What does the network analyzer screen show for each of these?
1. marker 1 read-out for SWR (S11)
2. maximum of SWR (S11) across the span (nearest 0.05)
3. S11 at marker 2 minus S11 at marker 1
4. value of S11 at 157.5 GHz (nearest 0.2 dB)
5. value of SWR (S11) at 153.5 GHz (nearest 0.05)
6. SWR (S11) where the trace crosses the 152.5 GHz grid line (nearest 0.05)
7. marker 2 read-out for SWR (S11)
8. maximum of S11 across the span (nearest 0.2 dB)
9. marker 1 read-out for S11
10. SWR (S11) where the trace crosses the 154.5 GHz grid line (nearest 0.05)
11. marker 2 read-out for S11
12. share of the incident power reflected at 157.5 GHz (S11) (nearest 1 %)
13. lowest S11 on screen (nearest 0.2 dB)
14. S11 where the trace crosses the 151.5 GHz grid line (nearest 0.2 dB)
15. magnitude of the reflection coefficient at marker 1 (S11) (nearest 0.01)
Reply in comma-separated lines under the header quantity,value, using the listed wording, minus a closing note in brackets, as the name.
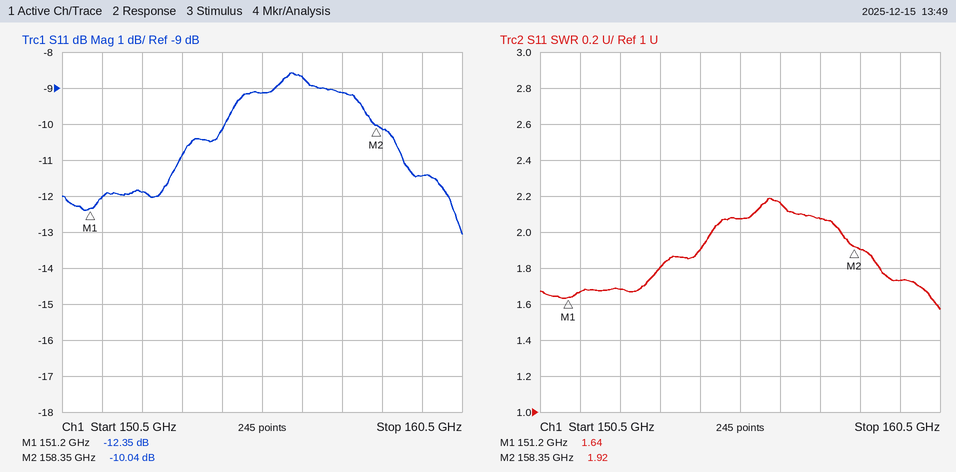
quantity,value
marker 1 read-out for SWR,1.64
maximum of SWR (S11) across the span,2.20
S11 at marker 2 minus S11 at marker 1,2.31 dB
value of S11 at 157.5 GHz,-9.2 dB
value of SWR (S11) at 153.5 GHz,1.80
SWR (S11) where the trace crosses the 152.5 GHz grid line,1.70
marker 2 read-out for SWR,1.92
maximum of S11 across the span,-8.6 dB
marker 1 read-out for S11,-12.35 dB
SWR (S11) where the trace crosses the 154.5 GHz grid line,1.90
marker 2 read-out for S11,-10.04 dB
share of the incident power reflected at 157.5 GHz (S11),12 %
lowest S11 on screen,-13.0 dB
S11 where the trace crosses the 151.5 GHz grid line,-12.0 dB
magnitude of the reflection coefficient at marker 1 (S11),0.24
